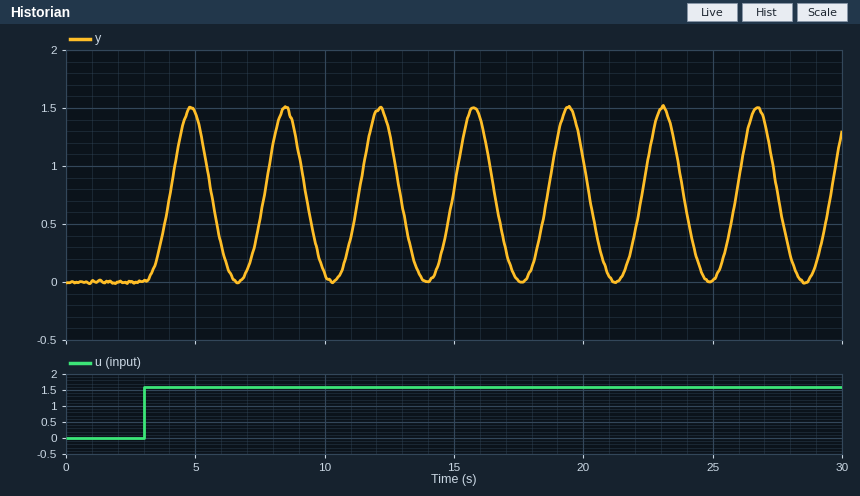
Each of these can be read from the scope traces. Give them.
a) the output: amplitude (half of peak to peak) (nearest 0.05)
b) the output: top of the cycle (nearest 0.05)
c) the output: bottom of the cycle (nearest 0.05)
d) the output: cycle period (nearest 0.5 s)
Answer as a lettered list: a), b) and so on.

a) 0.75
b) 1.50
c) 0.00
d) 3.5 s
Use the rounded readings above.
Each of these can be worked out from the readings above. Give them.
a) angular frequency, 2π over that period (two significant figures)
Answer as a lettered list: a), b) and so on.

a) 1.8 rad/s
